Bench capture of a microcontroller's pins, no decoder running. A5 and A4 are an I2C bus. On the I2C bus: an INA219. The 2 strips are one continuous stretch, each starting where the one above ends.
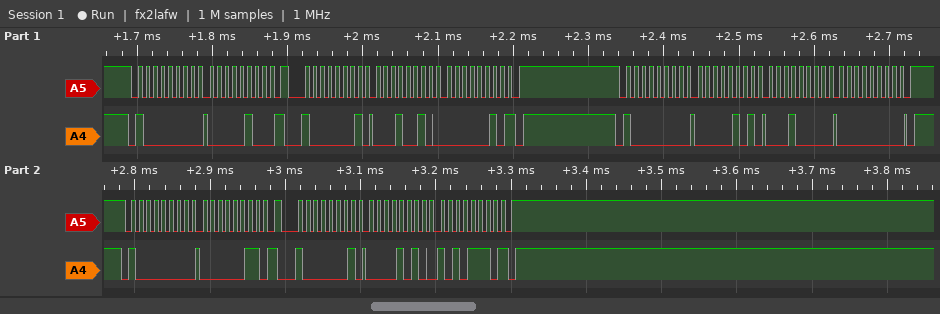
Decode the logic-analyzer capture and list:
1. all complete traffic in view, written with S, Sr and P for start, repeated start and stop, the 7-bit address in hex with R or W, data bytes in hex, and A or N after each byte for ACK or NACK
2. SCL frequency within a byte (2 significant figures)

S 40W A 04 A Sr 40R A 12 A 02 N P S 40W A 05 A 10 A 00 A P S 40W A 03 A Sr 40R A 0A A AE N P
100 kHz
